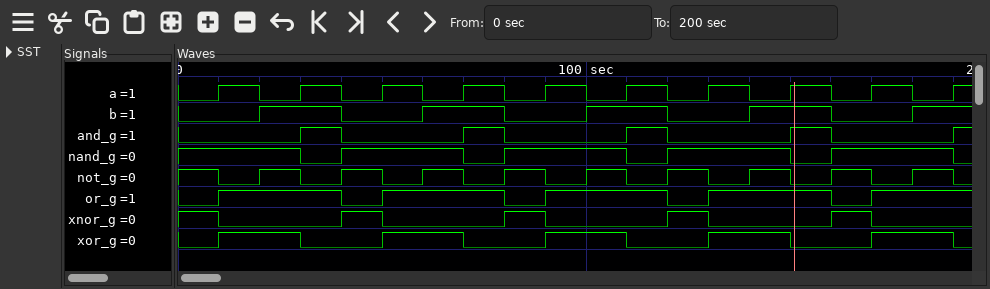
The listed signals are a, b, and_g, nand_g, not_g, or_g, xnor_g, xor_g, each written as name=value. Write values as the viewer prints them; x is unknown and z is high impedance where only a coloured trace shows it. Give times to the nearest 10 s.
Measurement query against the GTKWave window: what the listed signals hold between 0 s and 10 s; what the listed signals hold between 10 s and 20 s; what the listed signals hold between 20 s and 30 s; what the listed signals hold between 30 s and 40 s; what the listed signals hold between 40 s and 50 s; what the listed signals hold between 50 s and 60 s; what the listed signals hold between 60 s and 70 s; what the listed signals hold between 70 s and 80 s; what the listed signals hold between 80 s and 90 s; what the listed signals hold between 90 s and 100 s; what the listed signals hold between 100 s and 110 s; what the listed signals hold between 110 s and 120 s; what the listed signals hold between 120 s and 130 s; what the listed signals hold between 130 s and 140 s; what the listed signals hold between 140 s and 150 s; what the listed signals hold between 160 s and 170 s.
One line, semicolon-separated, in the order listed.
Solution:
a=0, b=0, and_g=0, nand_g=1, not_g=1, or_g=0, xnor_g=1, xor_g=0; a=1, b=0, and_g=0, nand_g=1, not_g=0, or_g=1, xnor_g=0, xor_g=1; a=0, b=1, and_g=0, nand_g=1, not_g=1, or_g=1, xnor_g=0, xor_g=1; a=1, b=1, and_g=1, nand_g=0, not_g=0, or_g=1, xnor_g=0, xor_g=0; a=0, b=0, and_g=0, nand_g=1, not_g=1, or_g=0, xnor_g=1, xor_g=0; a=1, b=0, and_g=0, nand_g=1, not_g=0, or_g=1, xnor_g=0, xor_g=1; a=0, b=1, and_g=0, nand_g=1, not_g=1, or_g=1, xnor_g=0, xor_g=1; a=1, b=1, and_g=1, nand_g=0, not_g=0, or_g=1, xnor_g=0, xor_g=0; a=0, b=0, and_g=0, nand_g=1, not_g=1, or_g=0, xnor_g=1, xor_g=0; a=1, b=0, and_g=0, nand_g=1, not_g=0, or_g=1, xnor_g=0, xor_g=1; a=0, b=1, and_g=0, nand_g=1, not_g=1, or_g=1, xnor_g=0, xor_g=1; a=1, b=1, and_g=1, nand_g=0, not_g=0, or_g=1, xnor_g=0, xor_g=0; a=0, b=0, and_g=0, nand_g=1, not_g=1, or_g=0, xnor_g=1, xor_g=0; a=1, b=0, and_g=0, nand_g=1, not_g=0, or_g=1, xnor_g=0, xor_g=1; a=0, b=1, and_g=0, nand_g=1, not_g=1, or_g=1, xnor_g=0, xor_g=1; a=0, b=0, and_g=0, nand_g=1, not_g=1, or_g=0, xnor_g=1, xor_g=0
